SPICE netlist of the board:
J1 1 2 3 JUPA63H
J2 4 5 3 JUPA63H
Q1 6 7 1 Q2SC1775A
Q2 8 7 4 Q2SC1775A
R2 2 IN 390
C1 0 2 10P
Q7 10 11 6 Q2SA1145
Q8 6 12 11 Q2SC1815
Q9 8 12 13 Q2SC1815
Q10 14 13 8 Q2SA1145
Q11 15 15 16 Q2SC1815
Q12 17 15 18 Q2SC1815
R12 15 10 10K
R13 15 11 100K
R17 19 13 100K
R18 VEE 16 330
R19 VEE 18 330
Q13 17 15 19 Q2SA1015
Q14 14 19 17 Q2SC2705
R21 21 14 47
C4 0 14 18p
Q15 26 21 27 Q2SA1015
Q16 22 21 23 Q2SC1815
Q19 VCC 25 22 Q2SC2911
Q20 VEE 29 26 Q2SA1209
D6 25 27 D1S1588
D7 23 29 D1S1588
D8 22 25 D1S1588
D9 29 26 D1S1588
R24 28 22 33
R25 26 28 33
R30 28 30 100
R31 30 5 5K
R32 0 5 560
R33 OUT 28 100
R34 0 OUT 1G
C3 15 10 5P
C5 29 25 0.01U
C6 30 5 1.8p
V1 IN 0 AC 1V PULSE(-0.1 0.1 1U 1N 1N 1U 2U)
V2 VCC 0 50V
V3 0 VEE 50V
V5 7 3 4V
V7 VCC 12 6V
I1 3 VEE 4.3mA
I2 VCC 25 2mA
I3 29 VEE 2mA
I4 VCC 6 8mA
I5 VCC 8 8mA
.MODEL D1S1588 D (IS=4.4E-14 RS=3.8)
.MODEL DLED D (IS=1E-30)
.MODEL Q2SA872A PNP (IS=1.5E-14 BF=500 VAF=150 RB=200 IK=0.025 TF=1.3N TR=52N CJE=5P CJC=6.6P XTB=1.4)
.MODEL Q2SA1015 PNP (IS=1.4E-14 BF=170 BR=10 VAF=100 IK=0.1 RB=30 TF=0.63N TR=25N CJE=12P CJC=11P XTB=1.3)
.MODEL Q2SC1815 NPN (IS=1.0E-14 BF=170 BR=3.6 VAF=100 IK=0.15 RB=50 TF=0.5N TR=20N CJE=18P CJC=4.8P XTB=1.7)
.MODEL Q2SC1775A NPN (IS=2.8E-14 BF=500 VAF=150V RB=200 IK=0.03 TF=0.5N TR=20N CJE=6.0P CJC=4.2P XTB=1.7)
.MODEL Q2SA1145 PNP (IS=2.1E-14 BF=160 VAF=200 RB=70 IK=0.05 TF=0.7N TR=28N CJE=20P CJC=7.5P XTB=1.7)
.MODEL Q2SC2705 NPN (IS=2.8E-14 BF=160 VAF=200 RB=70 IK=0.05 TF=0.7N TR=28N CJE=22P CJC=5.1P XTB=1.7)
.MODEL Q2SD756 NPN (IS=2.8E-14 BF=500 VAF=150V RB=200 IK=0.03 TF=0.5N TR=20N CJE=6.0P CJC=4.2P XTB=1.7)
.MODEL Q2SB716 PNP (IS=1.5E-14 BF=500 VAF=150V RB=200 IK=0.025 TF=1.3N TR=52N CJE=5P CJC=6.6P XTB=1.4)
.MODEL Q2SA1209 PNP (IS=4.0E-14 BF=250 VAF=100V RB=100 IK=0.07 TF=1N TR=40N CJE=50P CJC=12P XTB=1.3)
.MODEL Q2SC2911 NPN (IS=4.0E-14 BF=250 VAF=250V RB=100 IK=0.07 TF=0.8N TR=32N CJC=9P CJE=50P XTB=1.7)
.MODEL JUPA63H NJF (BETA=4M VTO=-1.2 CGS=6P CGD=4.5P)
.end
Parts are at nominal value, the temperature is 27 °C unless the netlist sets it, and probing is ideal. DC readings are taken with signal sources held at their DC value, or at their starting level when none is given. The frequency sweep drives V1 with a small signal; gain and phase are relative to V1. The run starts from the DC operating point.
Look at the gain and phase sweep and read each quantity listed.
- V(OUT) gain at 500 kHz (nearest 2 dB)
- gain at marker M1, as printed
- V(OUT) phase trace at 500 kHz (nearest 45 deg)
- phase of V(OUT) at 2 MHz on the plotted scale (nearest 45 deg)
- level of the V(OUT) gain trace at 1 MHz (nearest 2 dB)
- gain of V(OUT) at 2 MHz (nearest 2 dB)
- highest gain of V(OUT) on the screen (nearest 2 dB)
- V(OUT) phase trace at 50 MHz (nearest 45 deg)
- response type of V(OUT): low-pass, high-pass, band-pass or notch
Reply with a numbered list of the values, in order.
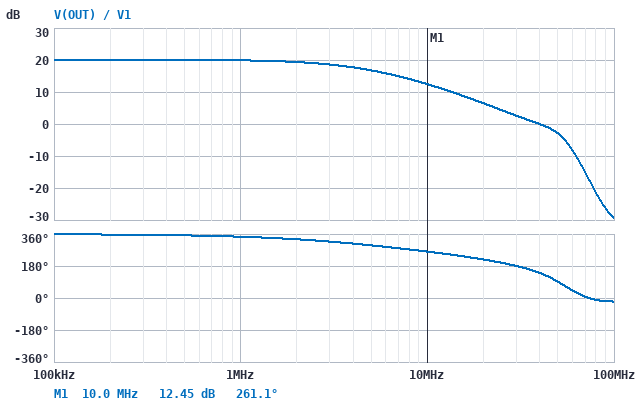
1. 20 dB
2. 12.45 dB
3. 360 deg
4. 315 deg
5. 20 dB
6. 20 dB
7. 20 dB
8. 90 deg
9. low-pass
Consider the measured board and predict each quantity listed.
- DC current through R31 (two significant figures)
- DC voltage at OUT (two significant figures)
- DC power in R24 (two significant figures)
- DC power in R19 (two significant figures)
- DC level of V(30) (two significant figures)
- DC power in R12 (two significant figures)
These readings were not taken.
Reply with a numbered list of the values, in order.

1. 160 µA
2. -910 mV
3. 11 mW
4. 11 mW
5. -890 mV
6. 250 mW
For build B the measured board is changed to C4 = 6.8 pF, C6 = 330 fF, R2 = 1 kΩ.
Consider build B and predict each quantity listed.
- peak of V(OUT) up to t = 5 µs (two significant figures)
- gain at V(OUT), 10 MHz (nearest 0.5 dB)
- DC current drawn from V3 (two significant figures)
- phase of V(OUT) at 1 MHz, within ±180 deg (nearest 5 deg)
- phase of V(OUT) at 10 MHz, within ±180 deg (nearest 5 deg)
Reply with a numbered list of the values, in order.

1. 1.2 V
2. 19.0 dB
3. 38 mA
4. -10 deg
5. -90 deg
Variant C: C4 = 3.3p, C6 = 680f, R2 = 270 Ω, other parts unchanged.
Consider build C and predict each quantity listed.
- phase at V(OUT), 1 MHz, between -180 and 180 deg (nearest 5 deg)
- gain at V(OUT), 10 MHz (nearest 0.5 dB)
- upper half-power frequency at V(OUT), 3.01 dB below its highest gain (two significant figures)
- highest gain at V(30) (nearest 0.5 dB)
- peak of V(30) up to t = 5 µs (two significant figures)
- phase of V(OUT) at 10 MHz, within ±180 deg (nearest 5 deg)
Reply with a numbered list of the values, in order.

1. -5 deg
2. 21.0 dB
3. 30 MHz
4. 24.5 dB
5. 1.8 V
6. -45 deg
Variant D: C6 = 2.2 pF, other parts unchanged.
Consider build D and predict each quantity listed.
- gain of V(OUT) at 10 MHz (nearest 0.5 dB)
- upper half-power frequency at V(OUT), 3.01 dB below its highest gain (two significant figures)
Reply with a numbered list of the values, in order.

1. 12.0 dB
2. 4.4 MHz
